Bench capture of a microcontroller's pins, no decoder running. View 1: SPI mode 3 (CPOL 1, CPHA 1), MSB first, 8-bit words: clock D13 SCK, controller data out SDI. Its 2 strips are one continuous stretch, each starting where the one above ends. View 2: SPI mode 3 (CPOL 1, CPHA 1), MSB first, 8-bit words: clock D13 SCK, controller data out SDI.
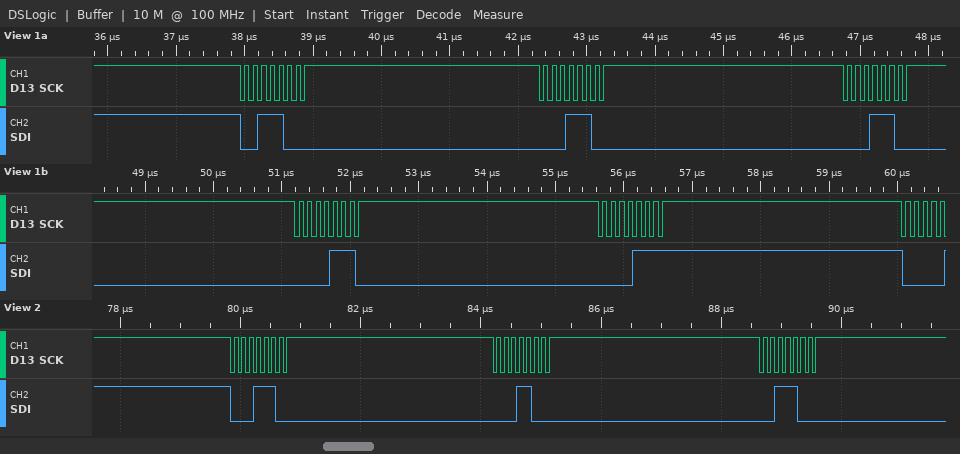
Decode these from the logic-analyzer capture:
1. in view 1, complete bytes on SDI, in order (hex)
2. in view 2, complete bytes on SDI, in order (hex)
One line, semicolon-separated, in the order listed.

38 1C 1C 0E 0F; 0x1C 0x18 0x38
